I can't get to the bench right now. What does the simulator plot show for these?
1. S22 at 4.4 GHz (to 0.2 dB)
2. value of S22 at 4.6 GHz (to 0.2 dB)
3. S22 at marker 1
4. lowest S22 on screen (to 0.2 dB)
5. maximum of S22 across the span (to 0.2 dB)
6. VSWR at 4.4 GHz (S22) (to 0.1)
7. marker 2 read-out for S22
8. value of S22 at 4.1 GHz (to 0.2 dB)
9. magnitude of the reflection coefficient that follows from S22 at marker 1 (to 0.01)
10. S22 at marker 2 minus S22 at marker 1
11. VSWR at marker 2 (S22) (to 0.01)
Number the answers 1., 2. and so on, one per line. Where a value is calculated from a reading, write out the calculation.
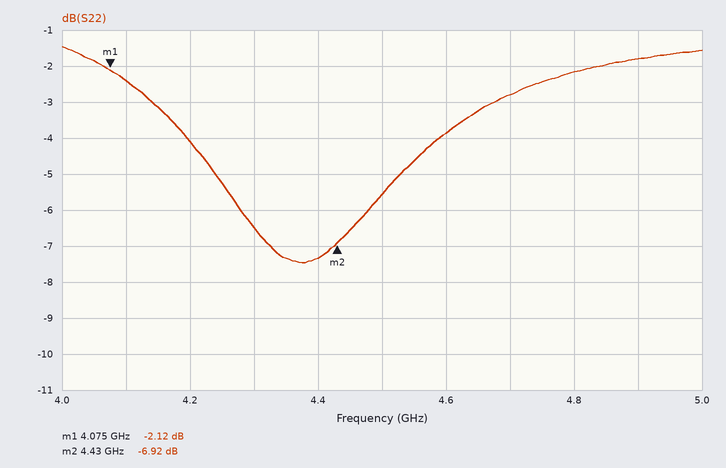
1. -7.4 dB
2. -3.8 dB
3. -2.12 dB
4. -7.4 dB
5. -1.4 dB
6. |Γ| = 10^(-7.4/20) = 0.4266; VSWR = (1 + 0.4266)/(1 − 0.4266) ≈ 2.5
7. -6.92 dB
8. -2.4 dB
9. 10^(-2.12/20) ≈ 0.78
10. -6.92 − (-2.12) = -4.80 dB
11. (1 + 0.4508)/(1 − 0.4508) ≈ 2.64
